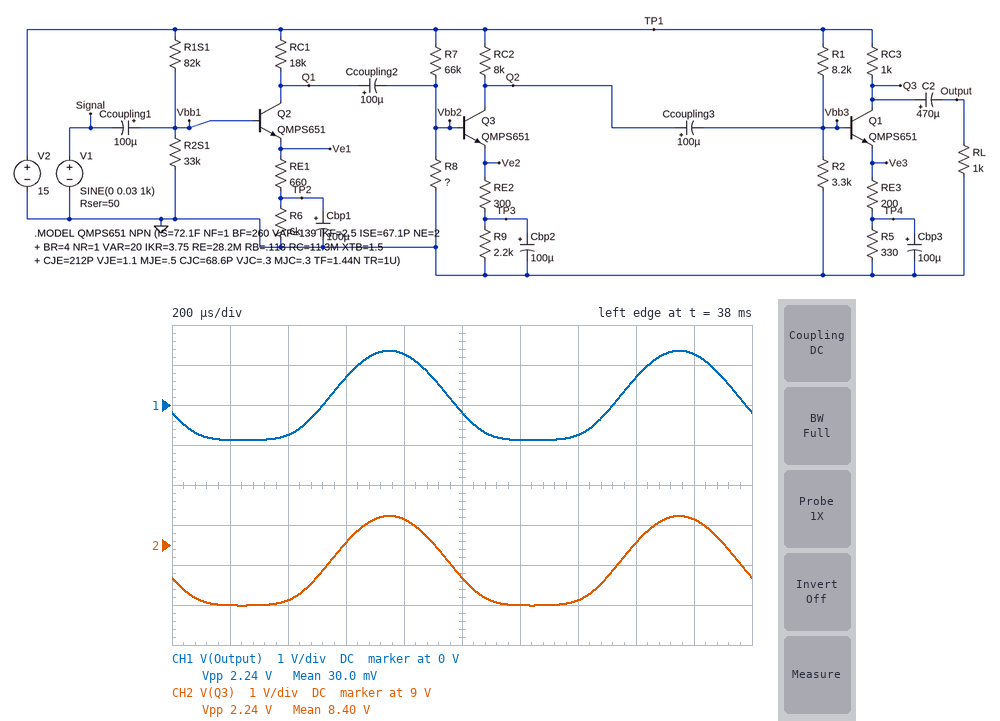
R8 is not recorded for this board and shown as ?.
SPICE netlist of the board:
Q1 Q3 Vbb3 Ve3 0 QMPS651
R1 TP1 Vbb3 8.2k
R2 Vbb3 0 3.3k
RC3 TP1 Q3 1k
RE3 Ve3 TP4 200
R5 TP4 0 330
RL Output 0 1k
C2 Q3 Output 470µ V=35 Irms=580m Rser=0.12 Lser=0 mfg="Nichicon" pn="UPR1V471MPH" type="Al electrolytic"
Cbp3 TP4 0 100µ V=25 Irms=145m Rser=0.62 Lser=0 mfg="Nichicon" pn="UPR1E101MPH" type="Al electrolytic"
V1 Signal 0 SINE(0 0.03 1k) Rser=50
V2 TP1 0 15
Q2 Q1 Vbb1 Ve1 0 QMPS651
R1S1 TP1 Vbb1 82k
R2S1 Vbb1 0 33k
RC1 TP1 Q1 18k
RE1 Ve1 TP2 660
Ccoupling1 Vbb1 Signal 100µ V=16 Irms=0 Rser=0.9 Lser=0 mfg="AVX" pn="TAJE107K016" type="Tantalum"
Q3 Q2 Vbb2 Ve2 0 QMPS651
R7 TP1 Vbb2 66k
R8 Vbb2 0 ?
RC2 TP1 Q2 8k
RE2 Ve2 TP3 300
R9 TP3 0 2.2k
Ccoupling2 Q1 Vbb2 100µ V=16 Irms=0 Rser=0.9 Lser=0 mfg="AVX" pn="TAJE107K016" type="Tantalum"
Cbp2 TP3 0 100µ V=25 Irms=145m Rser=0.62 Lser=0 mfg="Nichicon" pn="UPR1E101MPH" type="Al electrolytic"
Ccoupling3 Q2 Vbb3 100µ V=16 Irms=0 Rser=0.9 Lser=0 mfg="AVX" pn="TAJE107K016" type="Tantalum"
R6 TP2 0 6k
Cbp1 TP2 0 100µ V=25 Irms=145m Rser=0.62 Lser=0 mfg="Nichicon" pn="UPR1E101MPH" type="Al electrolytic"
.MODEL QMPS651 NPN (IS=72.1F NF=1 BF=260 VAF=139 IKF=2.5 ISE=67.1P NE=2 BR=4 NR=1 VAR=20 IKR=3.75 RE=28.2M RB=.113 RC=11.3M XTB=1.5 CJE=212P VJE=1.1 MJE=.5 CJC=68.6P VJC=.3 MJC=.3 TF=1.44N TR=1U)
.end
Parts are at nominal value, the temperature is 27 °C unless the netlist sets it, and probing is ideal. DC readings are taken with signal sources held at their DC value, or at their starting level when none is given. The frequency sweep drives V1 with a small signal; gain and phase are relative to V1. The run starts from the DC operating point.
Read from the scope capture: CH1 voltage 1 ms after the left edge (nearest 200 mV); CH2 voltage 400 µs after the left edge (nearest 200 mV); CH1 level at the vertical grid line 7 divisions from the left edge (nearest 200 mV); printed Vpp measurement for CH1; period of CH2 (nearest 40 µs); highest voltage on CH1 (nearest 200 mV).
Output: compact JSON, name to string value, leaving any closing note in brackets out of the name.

{"CH1 voltage 1 ms after the left edge": "-200 mV", "CH2 voltage 400 µs after the left edge": "7.6 V", "CH1 level at the vertical grid line 7 divisions from the left edge": "-800 mV", "printed Vpp measurement for CH1": "2.24 V", "period of CH2": "1.00 ms", "highest voltage on CH1": "1.4 V"}
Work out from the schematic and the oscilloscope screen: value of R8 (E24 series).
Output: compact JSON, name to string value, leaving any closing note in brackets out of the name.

{"value of R8": "5.1 kΩ"}
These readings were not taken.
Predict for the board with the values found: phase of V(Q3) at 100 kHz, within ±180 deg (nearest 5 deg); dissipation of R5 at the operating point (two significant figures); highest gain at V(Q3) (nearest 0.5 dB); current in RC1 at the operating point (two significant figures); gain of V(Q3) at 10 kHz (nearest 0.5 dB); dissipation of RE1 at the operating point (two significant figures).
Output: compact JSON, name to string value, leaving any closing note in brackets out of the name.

{"phase of V(Q3) at 100 kHz, within ±180 deg": "140 deg", "dissipation of R5 at the operating point": "15 mW", "highest gain at V(Q3)": "33.0 dB", "current in RC1 at the operating point": "520 µA", "gain of V(Q3) at 10 kHz": "33.0 dB", "dissipation of RE1 at the operating point": "190 µW"}
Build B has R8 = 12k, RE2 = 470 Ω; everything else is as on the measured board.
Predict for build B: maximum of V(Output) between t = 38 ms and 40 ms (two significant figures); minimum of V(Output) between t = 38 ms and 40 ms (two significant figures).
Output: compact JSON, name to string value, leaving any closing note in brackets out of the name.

{"maximum of V(Output) between t = 38 ms and 40 ms": "2.0 V", "minimum of V(Output) between t = 38 ms and 40 ms": "-1.9 V"}
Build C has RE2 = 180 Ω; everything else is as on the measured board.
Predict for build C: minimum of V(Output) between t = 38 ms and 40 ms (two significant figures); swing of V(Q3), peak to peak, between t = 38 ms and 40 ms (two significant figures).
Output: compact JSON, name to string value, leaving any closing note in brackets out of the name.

{"minimum of V(Output) between t = 38 ms and 40 ms": "-990 mV", "swing of V(Q3), peak to peak, between t = 38 ms and 40 ms": "2.8 V"}
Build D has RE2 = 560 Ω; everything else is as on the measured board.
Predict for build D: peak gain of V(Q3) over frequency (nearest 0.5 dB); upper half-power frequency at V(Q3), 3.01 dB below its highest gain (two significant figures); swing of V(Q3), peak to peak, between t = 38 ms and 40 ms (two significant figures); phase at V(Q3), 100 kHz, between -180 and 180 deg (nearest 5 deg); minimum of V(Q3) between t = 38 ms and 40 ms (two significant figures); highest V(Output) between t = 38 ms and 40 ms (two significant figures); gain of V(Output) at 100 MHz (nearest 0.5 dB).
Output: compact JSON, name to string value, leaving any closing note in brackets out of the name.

{"peak gain of V(Q3) over frequency": "29.0 dB", "upper half-power frequency at V(Q3), 3.01 dB below its highest gain": "200 kHz", "swing of V(Q3), peak to peak, between t = 38 ms and 40 ms": "1.6 V", "phase at V(Q3), 100 kHz, between -180 and 180 deg": "145 deg", "minimum of V(Q3) between t = 38 ms and 40 ms": "7.7 V", "highest V(Output) between t = 38 ms and 40 ms": "870 mV", "gain of V(Output) at 100 MHz": "-4.5 dB"}
